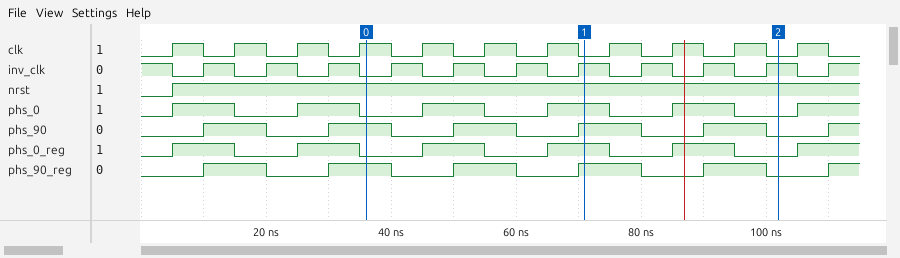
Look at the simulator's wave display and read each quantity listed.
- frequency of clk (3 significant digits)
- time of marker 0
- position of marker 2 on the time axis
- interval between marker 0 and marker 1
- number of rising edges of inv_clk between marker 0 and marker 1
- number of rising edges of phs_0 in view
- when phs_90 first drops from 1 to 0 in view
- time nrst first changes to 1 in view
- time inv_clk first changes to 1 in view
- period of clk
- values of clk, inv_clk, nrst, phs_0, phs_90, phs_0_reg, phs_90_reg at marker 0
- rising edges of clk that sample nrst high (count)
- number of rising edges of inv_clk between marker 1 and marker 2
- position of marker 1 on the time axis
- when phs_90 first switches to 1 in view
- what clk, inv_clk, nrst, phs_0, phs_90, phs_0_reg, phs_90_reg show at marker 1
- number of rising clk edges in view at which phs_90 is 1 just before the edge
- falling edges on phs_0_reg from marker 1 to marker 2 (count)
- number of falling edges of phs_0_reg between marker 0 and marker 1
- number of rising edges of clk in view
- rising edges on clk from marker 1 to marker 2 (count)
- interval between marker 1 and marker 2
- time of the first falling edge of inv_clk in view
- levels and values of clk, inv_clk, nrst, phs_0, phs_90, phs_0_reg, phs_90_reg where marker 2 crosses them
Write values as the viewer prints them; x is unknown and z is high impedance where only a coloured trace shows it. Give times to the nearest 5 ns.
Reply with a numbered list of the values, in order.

1. 100 MHz
2. 35 ns
3. 100 ns
4. 35 ns
5. 4
6. 6
7. 20 ns
8. 5 ns
9. 10 ns
10. 10 ns
11. clk=1, inv_clk=0, nrst=1, phs_0=0, phs_90=1, phs_0_reg=0, phs_90_reg=1
12. 10
13. 3
14. 70 ns
15. 10 ns
16. clk=0, inv_clk=1, nrst=1, phs_0=1, phs_90=1, phs_0_reg=1, phs_90_reg=1
17. 5
18. 2
19. 1
20. 11
21. 3
22. 30 ns
23. 5 ns
24. clk=0, inv_clk=1, nrst=1, phs_0=0, phs_90=0, phs_0_reg=0, phs_90_reg=0
